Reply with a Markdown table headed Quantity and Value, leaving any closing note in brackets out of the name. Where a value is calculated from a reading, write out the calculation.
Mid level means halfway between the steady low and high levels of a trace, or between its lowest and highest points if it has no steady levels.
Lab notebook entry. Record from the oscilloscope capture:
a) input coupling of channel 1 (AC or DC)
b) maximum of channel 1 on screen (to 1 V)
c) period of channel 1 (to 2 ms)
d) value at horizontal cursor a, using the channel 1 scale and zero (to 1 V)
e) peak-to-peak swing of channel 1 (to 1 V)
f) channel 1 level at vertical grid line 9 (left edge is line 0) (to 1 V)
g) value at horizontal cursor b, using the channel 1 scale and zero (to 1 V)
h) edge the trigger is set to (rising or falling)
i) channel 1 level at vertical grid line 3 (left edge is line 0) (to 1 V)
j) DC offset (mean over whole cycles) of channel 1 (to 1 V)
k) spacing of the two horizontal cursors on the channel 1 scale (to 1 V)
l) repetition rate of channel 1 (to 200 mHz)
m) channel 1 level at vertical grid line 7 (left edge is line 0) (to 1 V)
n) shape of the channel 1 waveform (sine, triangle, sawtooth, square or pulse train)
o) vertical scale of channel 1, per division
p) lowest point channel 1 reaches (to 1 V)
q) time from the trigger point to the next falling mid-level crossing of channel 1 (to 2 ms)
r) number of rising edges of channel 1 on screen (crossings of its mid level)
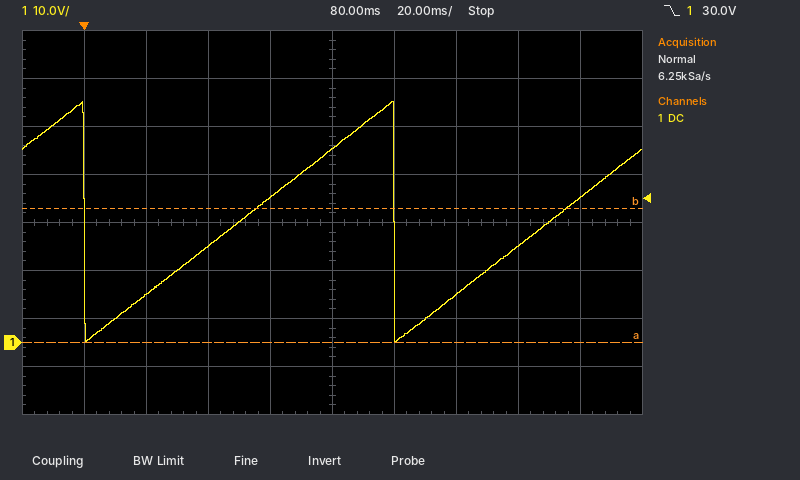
| Quantity | Value |
|---|---|
| input coupling of channel 1 | DC |
| maximum of channel 1 on screen | 50 V |
| period of channel 1 | 100 ms |
| value at horizontal cursor a, using the channel 1 scale and zero | 0 V |
| peak-to-peak swing of channel 1 | 50 V − (0 V) = 50 V |
| channel 1 level at vertical grid line 9 (left edge is line 0) | 30 V |
| value at horizontal cursor b, using the channel 1 scale and zero | 28 V |
| edge the trigger is set to | falling |
| channel 1 level at vertical grid line 3 (left edge is line 0) | 20 V |
| DC offset (mean over whole cycles) of channel 1 | (50 V + (0 V)) / 2 ≈ 25 V |
| spacing of the two horizontal cursors on the channel 1 scale | 28 V |
| repetition rate of channel 1 | 1 / 100 ms ≈ 10.0 Hz |
| channel 1 level at vertical grid line 7 (left edge is line 0) | 10 V |
| shape of the channel 1 waveform | sawtooth |
| vertical scale of channel 1, per division | 10 V |
| lowest point channel 1 reaches | 0 V |
| time from the trigger point to the next falling mid-level crossing of channel 1 | 100 ms |
| number of rising edges of channel 1 on screen | 2 |
